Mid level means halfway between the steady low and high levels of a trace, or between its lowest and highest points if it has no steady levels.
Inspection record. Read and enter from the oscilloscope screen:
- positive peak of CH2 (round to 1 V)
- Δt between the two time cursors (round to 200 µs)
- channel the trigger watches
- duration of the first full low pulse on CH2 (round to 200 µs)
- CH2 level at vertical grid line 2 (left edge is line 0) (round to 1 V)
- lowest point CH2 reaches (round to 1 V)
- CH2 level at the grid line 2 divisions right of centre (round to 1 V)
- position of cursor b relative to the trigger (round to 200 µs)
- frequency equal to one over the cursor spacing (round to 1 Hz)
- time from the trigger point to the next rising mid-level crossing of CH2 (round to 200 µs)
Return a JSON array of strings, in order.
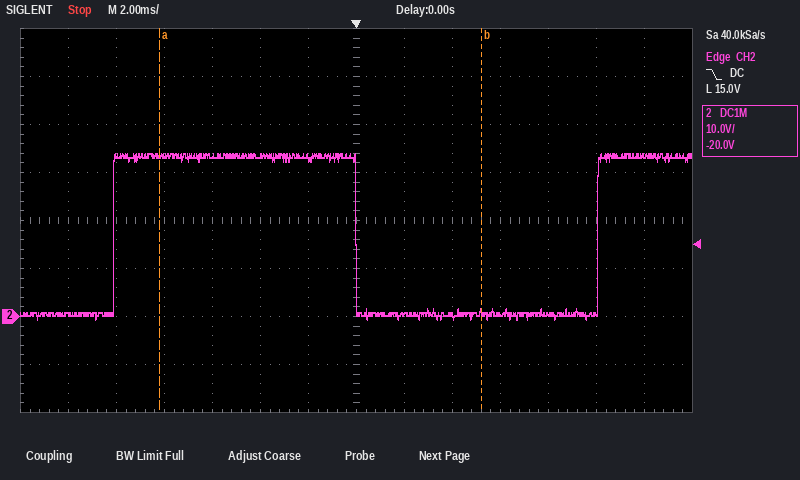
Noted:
["34 V", "13.4 ms", "CH2", "10.0 ms", "33 V", "-1 V", "0 V", "+5.2 ms", "75 Hz", "10.0 ms"]
